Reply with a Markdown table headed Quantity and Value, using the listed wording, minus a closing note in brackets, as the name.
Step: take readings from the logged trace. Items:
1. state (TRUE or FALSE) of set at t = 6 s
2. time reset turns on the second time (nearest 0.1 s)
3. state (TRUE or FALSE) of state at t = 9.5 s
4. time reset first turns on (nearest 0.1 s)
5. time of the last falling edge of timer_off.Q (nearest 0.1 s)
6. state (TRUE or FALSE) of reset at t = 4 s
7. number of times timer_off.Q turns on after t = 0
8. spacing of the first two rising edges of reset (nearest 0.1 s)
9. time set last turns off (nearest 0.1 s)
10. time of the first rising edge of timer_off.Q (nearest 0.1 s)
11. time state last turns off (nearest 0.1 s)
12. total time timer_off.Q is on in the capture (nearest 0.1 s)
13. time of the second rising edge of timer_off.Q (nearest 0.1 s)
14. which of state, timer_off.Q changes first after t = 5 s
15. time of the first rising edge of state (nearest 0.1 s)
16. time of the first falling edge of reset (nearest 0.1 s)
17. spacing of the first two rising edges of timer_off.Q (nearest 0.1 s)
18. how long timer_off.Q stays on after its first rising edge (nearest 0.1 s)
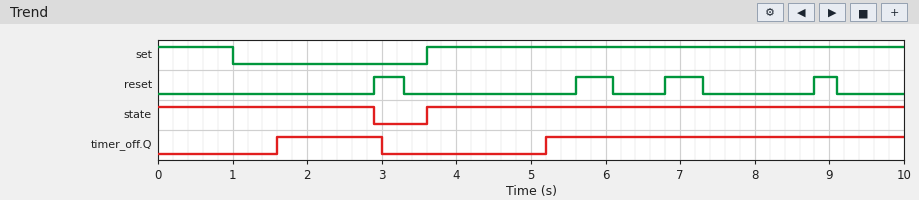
| Quantity | Value |
|---|---|
| state (TRUE or FALSE) of set at t = 6 s | TRUE |
| time reset turns on the second time | 5.6 s |
| state (TRUE or FALSE) of state at t = 9.5 s | TRUE |
| time reset first turns on | 2.9 s |
| time of the last falling edge of timer_off.Q | 3.0 s |
| state (TRUE or FALSE) of reset at t = 4 s | FALSE |
| number of times timer_off.Q turns on after t = 0 | 2 |
| spacing of the first two rising edges of reset | 2.7 s |
| time set last turns off | 1.0 s |
| time of the first rising edge of timer_off.Q | 1.6 s |
| time state last turns off | 2.9 s |
| total time timer_off.Q is on in the capture | 6.2 s |
| time of the second rising edge of timer_off.Q | 5.2 s |
| which of state, timer_off.Q changes first after t = 5 s | timer_off.Q |
| time of the first rising edge of state | 3.6 s |
| time of the first falling edge of reset | 3.3 s |
| spacing of the first two rising edges of timer_off.Q | 3.6 s |
| how long timer_off.Q stays on after its first rising edge | 1.4 s |
